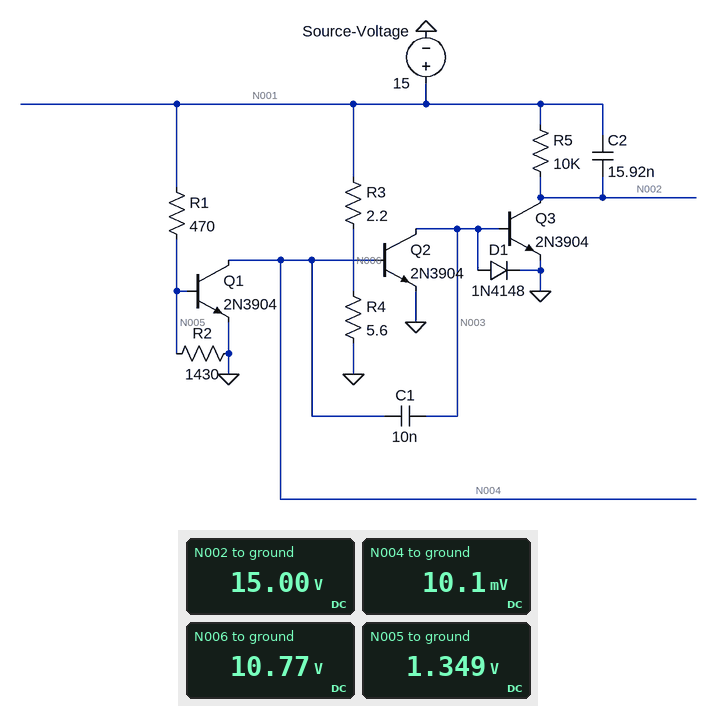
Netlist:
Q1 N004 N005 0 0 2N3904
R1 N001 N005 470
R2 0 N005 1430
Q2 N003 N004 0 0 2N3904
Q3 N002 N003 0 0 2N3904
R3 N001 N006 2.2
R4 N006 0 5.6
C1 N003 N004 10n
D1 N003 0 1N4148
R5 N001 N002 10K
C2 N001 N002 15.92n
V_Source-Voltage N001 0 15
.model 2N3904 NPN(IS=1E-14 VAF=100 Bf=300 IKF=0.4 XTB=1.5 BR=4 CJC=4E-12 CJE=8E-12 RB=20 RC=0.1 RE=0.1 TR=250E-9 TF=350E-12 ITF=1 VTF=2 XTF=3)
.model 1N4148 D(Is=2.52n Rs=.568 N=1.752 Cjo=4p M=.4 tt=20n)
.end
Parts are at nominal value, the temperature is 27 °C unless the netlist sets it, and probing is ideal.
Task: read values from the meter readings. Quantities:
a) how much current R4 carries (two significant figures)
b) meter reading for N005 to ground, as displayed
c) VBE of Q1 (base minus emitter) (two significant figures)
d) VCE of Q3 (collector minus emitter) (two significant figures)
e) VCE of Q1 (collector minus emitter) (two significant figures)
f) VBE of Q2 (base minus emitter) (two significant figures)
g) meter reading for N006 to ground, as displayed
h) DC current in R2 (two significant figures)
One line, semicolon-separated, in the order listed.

1.9 A; 1.349 V; 1.3 V; 15 V; 10 mV; 10 mV; 10.77 V; 940 µA
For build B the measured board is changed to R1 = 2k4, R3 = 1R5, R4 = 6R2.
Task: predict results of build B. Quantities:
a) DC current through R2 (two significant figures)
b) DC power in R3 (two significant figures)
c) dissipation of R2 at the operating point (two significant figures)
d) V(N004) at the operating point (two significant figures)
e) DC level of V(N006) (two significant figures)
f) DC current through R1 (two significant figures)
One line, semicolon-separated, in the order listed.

590 µA; 5.7 W; 500 µW; 6.7 mV; 12 V; 5.9 mA
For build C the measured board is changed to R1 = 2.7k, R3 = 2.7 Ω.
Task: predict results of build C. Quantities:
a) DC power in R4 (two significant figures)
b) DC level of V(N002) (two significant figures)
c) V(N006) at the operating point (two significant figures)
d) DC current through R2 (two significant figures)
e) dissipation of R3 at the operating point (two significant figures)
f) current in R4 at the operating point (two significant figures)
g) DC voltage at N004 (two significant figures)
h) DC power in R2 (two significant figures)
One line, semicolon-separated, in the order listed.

18 W; 15 V; 10 V; 580 µA; 8.8 W; 1.8 A; 6.6 mV; 480 µW
